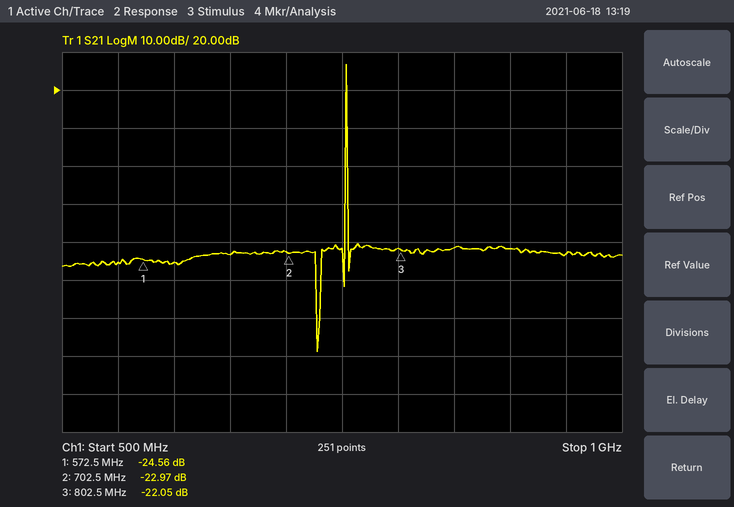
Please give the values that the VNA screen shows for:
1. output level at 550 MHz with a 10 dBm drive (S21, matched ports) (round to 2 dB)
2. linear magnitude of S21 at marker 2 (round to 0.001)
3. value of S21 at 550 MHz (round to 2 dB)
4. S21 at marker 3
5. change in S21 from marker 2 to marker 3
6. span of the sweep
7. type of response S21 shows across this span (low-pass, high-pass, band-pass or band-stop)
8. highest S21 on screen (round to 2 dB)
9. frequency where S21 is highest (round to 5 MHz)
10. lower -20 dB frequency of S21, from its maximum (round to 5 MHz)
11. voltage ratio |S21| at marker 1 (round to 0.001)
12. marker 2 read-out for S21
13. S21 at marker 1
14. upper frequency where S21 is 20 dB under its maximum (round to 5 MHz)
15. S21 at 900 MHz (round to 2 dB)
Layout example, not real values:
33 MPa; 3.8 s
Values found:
-16 dBm; 0.071; -26 dB; -22.05 dB; 0.92 dB; 500 MHz; band-pass; 26 dB; 755 MHz; 755 MHz; 0.059; -22.97 dB; -24.56 dB; 755 MHz; -22 dB
